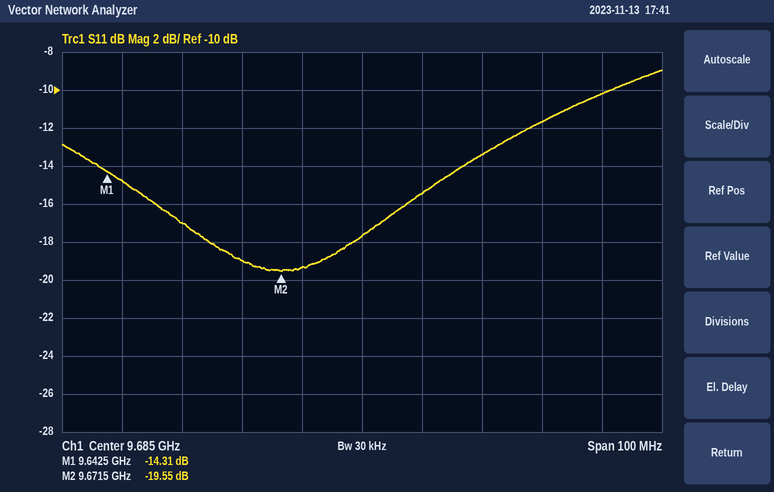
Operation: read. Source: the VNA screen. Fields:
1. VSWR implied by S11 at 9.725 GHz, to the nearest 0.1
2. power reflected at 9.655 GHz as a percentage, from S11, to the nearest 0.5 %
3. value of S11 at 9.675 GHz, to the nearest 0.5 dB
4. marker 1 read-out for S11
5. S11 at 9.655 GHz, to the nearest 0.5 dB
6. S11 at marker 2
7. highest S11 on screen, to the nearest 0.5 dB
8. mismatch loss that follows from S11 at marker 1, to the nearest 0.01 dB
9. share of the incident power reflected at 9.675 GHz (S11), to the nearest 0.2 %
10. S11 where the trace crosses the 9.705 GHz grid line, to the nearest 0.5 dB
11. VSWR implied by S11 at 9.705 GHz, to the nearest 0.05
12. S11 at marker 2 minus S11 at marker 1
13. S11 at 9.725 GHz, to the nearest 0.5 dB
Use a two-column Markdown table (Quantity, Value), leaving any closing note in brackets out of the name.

| Quantity | Value |
|---|---|
| VSWR implied by S11 at 9.725 GHz, to the nearest 0.1 | 1.9 |
| power reflected at 9.655 GHz as a percentage, from S11, to the nearest 0.5 % | 2.0 % |
| value of S11 at 9.675 GHz, to the nearest 0.5 dB | -19.5 dB |
| marker 1 read-out for S11 | -14.31 dB |
| S11 at 9.655 GHz, to the nearest 0.5 dB | -17.0 dB |
| S11 at marker 2 | -19.55 dB |
| highest S11 on screen, to the nearest 0.5 dB | -9.0 dB |
| mismatch loss that follows from S11 at marker 1, to the nearest 0.01 dB | 0.16 dB |
| share of the incident power reflected at 9.675 GHz (S11), to the nearest 0.2 % | 1.2 % |
| S11 where the trace crosses the 9.705 GHz grid line, to the nearest 0.5 dB | -13.5 dB |
| VSWR implied by S11 at 9.705 GHz, to the nearest 0.05 | 1.55 |
| S11 at marker 2 minus S11 at marker 1 | -5.24 dB |
| S11 at 9.725 GHz, to the nearest 0.5 dB | -10.0 dB |
